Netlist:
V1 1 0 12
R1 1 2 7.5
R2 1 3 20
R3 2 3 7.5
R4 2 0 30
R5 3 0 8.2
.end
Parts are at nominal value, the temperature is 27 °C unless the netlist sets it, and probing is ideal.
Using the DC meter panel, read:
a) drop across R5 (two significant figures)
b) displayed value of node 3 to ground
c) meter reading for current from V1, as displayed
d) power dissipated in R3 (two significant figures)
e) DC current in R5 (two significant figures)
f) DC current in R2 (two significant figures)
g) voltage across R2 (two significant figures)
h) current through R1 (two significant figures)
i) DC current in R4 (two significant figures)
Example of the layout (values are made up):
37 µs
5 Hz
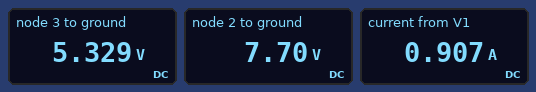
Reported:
5.3 V
5.329 V
0.907 A
750 mW
650 mA
330 mA
6.7 V
570 mA
260 mA
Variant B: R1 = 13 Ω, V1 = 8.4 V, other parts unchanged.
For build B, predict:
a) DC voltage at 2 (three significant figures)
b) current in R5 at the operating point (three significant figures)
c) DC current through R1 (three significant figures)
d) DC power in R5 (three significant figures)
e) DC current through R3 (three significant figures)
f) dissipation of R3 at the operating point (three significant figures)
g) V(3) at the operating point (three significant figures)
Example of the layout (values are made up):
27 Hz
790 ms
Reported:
4.48 V
406 mA
302 mA
1.35 W
153 mA
175 mW
3.33 V
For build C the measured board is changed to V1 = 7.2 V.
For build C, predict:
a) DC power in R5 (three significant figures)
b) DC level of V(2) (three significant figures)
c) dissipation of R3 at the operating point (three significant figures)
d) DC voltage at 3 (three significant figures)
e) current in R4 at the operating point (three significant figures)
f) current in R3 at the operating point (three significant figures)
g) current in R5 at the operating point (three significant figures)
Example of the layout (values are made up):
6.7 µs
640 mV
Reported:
1.25 W
4.62 V
270 mW
3.20 V
154 mA
190 mA
390 mA
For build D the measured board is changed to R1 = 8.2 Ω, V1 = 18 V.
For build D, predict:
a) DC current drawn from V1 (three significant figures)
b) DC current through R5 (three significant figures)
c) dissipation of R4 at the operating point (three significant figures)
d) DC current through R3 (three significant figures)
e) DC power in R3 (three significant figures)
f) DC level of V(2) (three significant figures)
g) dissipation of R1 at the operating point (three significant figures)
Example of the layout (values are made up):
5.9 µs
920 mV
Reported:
1.33 A
958 mA
4.21 W
451 mA
1.52 W
11.2 V
5.58 W
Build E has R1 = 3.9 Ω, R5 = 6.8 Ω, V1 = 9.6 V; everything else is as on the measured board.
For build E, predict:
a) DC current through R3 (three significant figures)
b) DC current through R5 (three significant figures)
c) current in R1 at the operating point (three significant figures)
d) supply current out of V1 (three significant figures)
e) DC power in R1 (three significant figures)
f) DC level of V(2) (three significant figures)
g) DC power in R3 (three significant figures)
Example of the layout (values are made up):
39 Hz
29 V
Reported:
378 mA
640 mA
618 mA
880 mA
1.49 W
7.19 V
1.07 W
